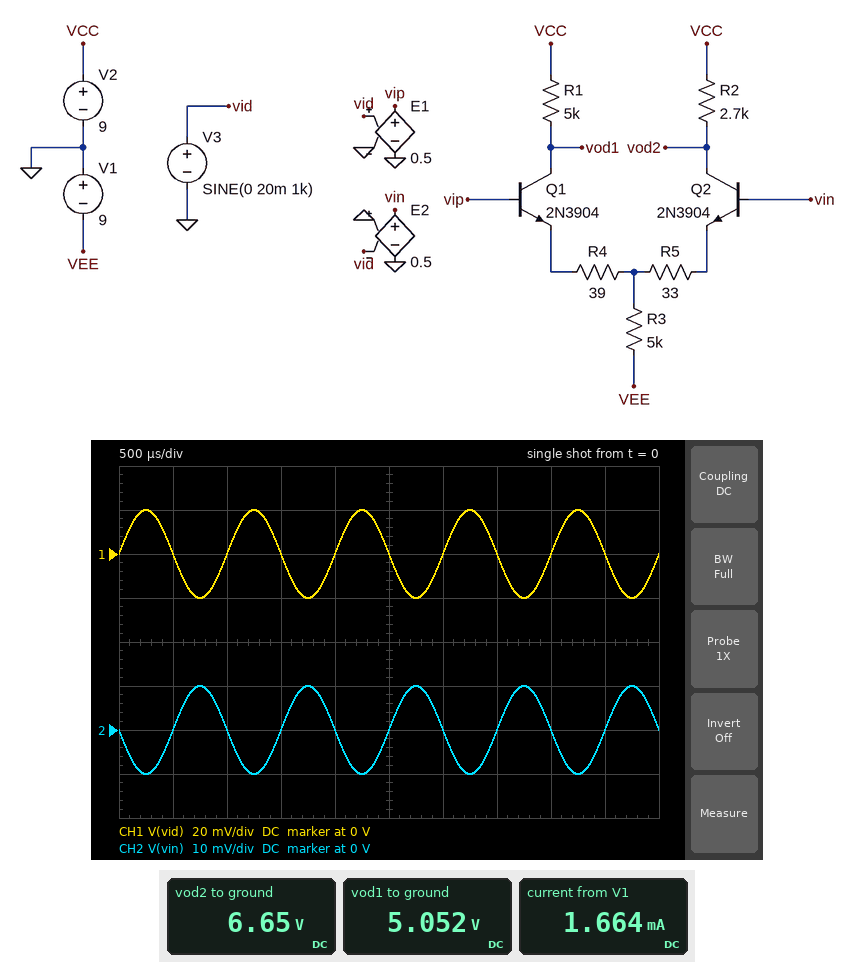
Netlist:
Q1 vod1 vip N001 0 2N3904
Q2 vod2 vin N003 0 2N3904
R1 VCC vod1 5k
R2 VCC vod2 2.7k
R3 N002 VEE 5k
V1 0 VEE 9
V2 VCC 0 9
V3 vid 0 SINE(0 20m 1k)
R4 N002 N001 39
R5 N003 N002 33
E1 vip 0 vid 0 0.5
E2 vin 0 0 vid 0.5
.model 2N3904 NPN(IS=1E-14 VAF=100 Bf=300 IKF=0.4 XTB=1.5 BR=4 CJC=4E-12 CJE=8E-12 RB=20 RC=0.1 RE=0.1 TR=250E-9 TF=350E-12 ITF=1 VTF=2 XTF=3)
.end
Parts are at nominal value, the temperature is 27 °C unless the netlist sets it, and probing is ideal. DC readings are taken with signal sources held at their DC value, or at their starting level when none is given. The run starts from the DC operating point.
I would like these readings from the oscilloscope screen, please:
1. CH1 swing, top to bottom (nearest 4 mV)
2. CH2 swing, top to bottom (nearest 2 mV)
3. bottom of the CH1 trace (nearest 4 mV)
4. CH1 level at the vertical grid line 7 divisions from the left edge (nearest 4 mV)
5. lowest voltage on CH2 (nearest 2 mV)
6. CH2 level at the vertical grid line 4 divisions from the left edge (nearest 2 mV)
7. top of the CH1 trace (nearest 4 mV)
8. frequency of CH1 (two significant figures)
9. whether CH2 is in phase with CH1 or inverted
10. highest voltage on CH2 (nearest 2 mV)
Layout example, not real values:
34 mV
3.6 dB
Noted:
40 mV
20 mV
-20 mV
0 V
-10 mV
0 V
20 mV
1.0 kHz
inverted
10 mV
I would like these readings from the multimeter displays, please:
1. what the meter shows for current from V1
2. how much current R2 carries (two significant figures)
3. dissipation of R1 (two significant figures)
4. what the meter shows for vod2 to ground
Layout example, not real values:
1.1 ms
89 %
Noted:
1.664 mA
870 µA
3.1 mW
6.65 V
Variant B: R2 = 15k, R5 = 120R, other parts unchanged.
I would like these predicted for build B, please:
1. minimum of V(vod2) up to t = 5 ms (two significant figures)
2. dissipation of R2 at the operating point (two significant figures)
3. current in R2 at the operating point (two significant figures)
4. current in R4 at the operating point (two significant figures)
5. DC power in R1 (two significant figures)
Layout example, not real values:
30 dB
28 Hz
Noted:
-170 mV
4.2 mW
530 µA
1.1 mA
6.4 mW
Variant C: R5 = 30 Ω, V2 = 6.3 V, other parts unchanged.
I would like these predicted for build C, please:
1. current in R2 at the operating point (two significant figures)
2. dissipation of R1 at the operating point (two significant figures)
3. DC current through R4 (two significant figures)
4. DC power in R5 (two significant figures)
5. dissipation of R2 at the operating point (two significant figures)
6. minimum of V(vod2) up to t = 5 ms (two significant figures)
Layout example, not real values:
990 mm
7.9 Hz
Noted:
890 µA
3.0 mW
770 µA
24 µW
2.1 mW
3.5 V
